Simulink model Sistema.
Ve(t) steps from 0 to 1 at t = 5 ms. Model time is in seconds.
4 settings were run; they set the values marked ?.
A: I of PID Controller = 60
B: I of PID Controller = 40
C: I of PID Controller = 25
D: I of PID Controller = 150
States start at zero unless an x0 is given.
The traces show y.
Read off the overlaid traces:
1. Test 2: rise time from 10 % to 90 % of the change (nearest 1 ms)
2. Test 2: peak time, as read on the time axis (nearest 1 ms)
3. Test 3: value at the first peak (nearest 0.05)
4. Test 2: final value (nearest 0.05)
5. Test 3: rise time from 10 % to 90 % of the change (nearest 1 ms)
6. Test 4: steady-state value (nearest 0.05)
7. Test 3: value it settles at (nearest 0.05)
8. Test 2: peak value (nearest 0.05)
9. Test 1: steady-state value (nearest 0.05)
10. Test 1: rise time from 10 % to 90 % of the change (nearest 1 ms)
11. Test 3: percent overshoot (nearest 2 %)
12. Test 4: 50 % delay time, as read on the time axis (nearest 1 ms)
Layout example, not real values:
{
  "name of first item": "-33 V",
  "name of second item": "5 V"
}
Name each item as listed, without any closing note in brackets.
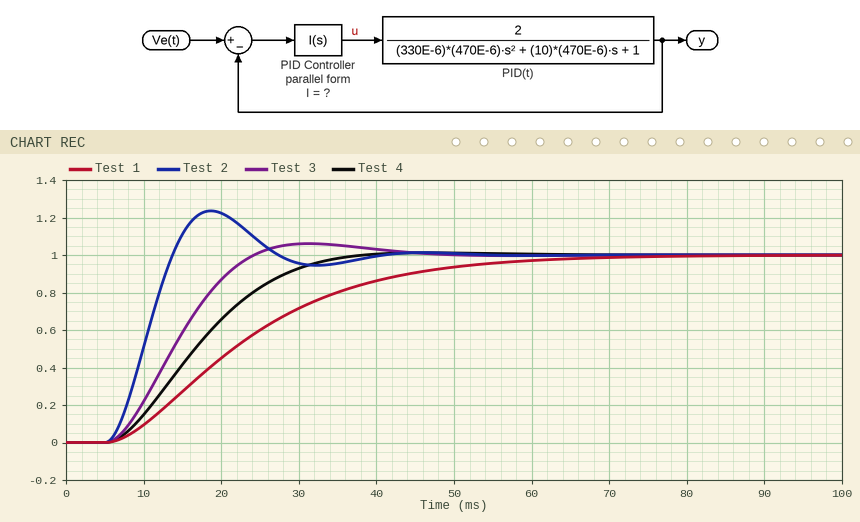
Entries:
{
  "Test 2: rise time from 10 % to 90 % of the change": "6 ms",
  "Test 2: peak time, as read on the time axis": "19 ms",
  "Test 3: value at the first peak": "1.05",
  "Test 2: final value": "1.00",
  "Test 3: rise time from 10 % to 90 % of the change": "13 ms",
  "Test 4: steady-state value": "1.00",
  "Test 3: value it settles at": "1.00",
  "Test 2: peak value": "1.25",
  "Test 1: steady-state value": "1.00",
  "Test 1: rise time from 10 % to 90 % of the change": "34 ms",
  "Test 3: percent overshoot": "6 %",
  "Test 4: 50 % delay time, as read on the time axis": "17 ms"
}
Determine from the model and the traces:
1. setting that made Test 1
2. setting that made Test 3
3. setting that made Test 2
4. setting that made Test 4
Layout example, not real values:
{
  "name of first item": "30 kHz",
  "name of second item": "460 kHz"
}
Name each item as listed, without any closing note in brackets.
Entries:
{
  "setting that made Test 1": "C",
  "setting that made Test 3": "A",
  "setting that made Test 2": "D",
  "setting that made Test 4": "B"
}
